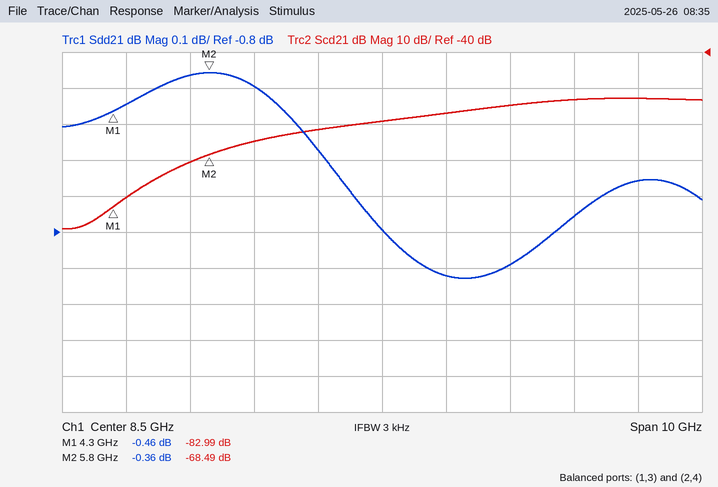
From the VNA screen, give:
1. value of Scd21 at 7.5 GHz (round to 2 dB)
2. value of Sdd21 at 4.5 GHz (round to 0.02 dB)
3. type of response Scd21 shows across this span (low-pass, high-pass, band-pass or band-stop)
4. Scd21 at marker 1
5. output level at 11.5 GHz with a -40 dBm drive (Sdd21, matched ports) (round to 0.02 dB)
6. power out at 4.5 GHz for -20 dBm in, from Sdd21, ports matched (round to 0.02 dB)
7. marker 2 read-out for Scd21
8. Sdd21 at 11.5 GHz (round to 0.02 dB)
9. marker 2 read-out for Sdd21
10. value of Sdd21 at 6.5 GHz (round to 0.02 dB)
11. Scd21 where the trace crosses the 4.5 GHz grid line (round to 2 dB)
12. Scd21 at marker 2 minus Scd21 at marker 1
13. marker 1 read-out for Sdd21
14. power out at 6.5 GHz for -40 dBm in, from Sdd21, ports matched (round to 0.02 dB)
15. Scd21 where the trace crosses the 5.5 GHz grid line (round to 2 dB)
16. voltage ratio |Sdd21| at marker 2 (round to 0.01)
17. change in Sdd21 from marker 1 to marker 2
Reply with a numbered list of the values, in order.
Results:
1. -62 dB
2. -0.44 dB
3. high-pass
4. -82.99 dB
5. -40.76 dBm
6. -20.44 dBm
7. -68.49 dB
8. -0.76 dB
9. -0.36 dB
10. -0.40 dB
11. -80 dB
12. 14.50 dB
13. -0.46 dB
14. -40.40 dBm
15. -70 dB
16. 0.96
17. 0.10 dB
